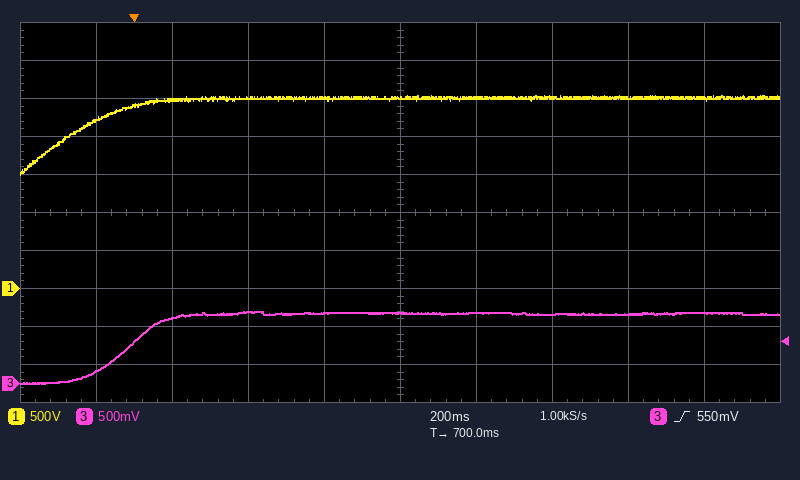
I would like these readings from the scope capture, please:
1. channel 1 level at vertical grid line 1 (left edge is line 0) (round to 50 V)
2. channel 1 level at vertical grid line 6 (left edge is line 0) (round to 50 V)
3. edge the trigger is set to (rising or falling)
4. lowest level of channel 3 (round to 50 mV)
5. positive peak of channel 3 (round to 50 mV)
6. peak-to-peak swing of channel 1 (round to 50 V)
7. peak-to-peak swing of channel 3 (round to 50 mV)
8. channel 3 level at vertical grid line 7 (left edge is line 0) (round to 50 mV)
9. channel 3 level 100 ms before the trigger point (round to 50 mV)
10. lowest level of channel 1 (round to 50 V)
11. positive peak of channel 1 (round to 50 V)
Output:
2.20 kV
2.50 kV
rising
0 mV
950 mV
1.05 kV
950 mV
900 mV
150 mV
1.50 kV
2.55 kV
